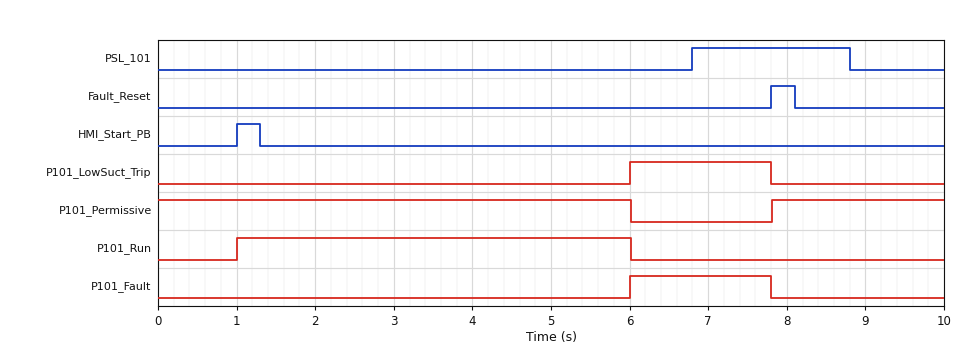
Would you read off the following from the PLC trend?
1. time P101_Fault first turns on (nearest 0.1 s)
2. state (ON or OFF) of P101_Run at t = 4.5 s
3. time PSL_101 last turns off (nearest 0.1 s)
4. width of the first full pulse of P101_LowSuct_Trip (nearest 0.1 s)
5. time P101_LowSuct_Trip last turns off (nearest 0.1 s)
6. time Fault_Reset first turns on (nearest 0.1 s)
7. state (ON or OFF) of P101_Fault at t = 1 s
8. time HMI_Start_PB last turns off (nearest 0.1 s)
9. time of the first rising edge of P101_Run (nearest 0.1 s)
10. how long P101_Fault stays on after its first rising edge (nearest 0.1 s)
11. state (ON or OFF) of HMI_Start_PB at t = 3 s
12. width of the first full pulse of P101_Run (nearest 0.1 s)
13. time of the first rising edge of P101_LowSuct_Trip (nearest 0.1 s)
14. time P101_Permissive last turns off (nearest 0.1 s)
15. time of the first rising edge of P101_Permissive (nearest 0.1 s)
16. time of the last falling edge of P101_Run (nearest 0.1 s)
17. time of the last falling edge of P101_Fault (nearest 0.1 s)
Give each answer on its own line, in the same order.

6.0 s
ON
8.8 s
1.8 s
7.8 s
7.8 s
OFF
1.3 s
1.0 s
1.8 s
OFF
5.0 s
6.0 s
6.0 s
7.8 s
6.0 s
7.8 s
